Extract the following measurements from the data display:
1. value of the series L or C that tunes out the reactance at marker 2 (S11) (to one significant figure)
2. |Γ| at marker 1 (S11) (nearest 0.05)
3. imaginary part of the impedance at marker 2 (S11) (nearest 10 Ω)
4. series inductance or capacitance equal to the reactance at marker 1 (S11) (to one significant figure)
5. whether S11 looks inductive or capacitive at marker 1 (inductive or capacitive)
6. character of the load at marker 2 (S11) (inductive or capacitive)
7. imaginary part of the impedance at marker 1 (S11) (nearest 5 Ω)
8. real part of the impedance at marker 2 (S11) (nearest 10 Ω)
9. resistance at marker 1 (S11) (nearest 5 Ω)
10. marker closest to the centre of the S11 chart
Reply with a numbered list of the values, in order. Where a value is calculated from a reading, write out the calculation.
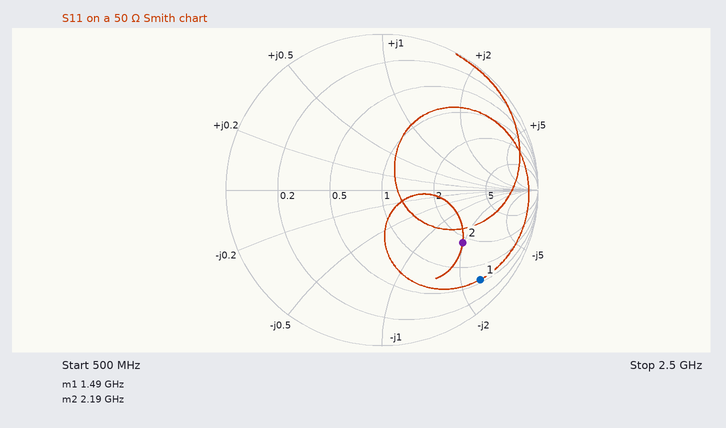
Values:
1. L = 100 Ω/(2π × 2.19 GHz) ≈ 7 nH
2. 0.85
3. -100 Ω
4. C = 1/(2π × 1.49 GHz × 125 Ω) ≈ 855 fF, so 900 fF to one significant figure
5. capacitive
6. capacitive
7. -125 Ω
8. 90 Ω
9. 30 Ω
10. marker 2
